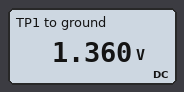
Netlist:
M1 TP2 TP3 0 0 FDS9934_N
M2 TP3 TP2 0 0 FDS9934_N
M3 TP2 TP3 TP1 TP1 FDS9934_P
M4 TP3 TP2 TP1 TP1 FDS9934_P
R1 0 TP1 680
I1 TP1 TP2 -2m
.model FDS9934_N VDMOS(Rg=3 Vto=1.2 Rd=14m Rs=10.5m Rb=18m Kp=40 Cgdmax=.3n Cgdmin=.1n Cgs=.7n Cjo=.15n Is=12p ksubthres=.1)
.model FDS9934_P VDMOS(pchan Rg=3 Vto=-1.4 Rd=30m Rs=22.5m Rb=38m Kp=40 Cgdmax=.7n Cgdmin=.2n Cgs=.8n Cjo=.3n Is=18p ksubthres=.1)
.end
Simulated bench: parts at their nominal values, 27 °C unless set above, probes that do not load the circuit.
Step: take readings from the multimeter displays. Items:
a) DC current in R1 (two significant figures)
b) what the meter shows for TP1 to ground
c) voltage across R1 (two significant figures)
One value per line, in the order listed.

2.0 mA
1.360 V
1.4 V
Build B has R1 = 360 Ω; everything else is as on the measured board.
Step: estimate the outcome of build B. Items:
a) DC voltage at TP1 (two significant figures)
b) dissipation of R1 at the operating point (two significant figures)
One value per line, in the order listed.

720 mV
1.4 mW
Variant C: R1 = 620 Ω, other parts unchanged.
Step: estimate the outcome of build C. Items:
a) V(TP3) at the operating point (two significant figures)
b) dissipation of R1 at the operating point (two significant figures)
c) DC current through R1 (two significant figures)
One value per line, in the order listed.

1.2 V
2.5 mW
2.0 mA
